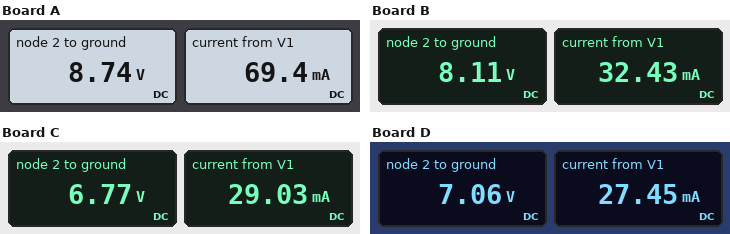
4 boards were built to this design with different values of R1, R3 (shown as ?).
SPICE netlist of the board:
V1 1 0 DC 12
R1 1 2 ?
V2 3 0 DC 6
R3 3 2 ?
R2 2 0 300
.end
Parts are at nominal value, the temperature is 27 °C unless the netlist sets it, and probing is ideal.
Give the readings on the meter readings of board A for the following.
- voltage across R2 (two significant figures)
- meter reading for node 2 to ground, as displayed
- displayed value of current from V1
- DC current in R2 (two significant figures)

8.7 V
8.74 V
69.4 mA
29 mA
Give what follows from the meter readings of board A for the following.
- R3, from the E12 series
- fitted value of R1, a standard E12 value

68 Ω
47 Ω
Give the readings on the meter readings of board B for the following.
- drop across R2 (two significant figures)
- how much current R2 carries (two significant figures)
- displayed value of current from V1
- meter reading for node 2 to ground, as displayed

8.1 V
27 mA
32.43 mA
8.11 V
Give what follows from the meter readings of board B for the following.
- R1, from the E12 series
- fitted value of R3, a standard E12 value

120 Ω
390 Ω
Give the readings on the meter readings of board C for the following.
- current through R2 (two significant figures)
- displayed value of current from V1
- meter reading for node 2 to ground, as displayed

23 mA
29.03 mA
6.77 V
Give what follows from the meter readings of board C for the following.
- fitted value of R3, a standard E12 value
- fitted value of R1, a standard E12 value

120 Ω
180 Ω
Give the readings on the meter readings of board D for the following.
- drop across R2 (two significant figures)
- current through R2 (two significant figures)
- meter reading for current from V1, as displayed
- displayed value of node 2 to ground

7.1 V
24 mA
27.45 mA
7.06 V
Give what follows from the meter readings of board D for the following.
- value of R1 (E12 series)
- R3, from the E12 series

180 Ω
270 Ω
